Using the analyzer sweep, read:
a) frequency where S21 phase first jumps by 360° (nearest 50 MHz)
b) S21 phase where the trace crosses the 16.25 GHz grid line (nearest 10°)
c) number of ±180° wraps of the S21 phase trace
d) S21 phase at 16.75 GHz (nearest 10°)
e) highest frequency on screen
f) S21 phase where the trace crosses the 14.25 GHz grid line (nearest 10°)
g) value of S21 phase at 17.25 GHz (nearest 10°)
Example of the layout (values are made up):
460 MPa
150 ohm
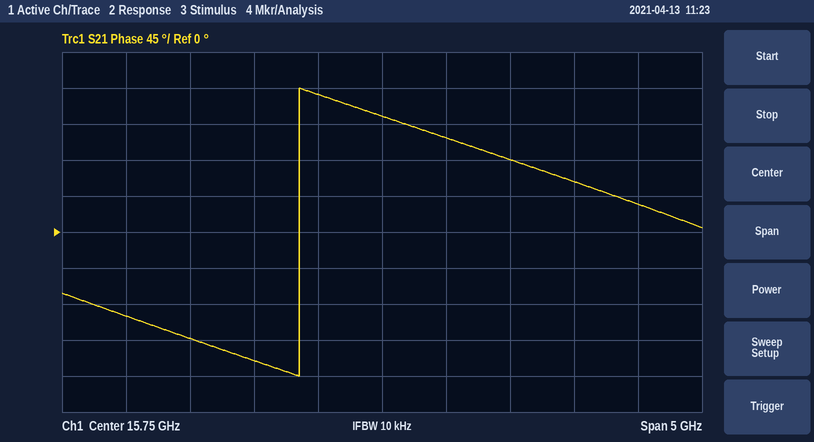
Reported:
15.10 GHz
120°
1
90°
18.25 GHz
-130°
60°
